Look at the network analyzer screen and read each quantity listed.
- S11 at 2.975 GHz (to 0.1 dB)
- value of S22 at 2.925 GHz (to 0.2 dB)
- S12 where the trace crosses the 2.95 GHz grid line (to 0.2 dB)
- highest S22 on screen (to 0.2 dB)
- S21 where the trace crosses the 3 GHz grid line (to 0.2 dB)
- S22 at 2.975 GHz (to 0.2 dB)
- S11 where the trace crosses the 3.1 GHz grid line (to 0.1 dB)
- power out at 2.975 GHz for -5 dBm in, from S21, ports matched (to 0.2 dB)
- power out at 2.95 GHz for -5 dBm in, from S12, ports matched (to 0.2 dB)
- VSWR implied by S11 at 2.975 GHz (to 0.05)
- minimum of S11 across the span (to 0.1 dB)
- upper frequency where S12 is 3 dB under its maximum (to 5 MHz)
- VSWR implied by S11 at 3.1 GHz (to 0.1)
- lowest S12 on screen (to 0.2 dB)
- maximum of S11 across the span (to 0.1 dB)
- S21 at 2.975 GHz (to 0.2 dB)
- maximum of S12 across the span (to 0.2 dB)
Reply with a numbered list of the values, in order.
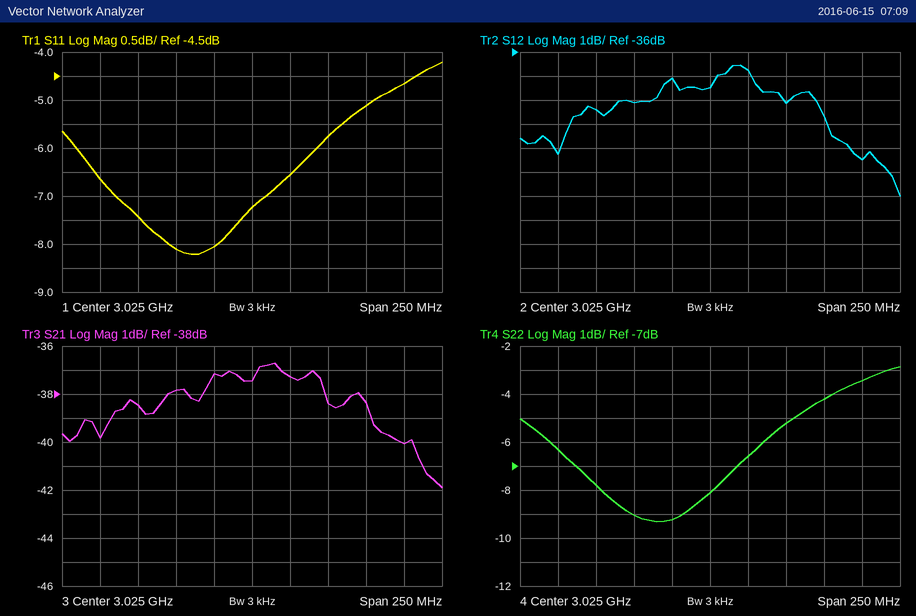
1. -8.1 dB
2. -6.4 dB
3. -38.4 dB
4. -2.8 dB
5. -37.2 dB
6. -9.0 dB
7. -5.1 dB
8. -42.8 dBm
9. -43.4 dBm
10. 2.30
11. -8.2 dB
12. 3.105 GHz
13. 3.5
14. -42.0 dB
15. -4.2 dB
16. -37.8 dB
17. -36.6 dB
